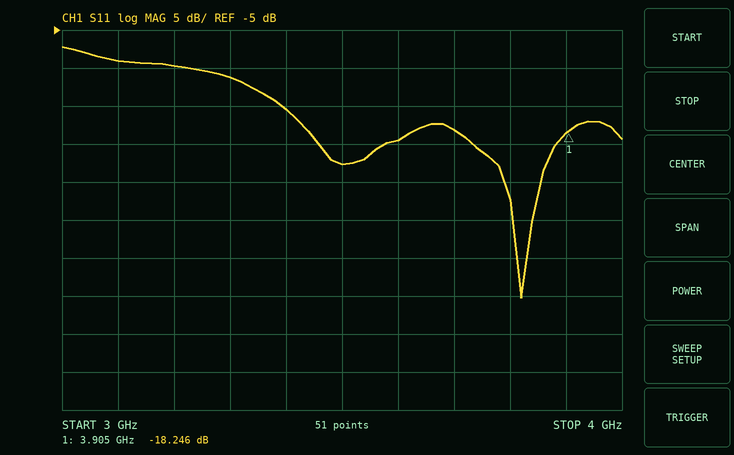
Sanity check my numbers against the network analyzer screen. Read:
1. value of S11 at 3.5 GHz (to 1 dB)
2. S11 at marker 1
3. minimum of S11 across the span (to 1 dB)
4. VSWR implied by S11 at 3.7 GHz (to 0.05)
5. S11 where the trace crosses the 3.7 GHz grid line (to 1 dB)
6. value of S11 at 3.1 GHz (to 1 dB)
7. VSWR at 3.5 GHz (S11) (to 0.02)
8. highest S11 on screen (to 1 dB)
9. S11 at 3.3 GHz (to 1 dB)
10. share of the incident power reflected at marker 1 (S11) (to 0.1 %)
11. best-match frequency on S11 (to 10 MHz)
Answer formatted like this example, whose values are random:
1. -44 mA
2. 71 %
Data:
1. -23 dB
2. -18.246 dB
3. -40 dB
4. 1.30
5. -18 dB
6. -9 dB
7. 1.16
8. -7 dB
9. -11 dB
10. 1.5 %
11. 3.82 GHz
